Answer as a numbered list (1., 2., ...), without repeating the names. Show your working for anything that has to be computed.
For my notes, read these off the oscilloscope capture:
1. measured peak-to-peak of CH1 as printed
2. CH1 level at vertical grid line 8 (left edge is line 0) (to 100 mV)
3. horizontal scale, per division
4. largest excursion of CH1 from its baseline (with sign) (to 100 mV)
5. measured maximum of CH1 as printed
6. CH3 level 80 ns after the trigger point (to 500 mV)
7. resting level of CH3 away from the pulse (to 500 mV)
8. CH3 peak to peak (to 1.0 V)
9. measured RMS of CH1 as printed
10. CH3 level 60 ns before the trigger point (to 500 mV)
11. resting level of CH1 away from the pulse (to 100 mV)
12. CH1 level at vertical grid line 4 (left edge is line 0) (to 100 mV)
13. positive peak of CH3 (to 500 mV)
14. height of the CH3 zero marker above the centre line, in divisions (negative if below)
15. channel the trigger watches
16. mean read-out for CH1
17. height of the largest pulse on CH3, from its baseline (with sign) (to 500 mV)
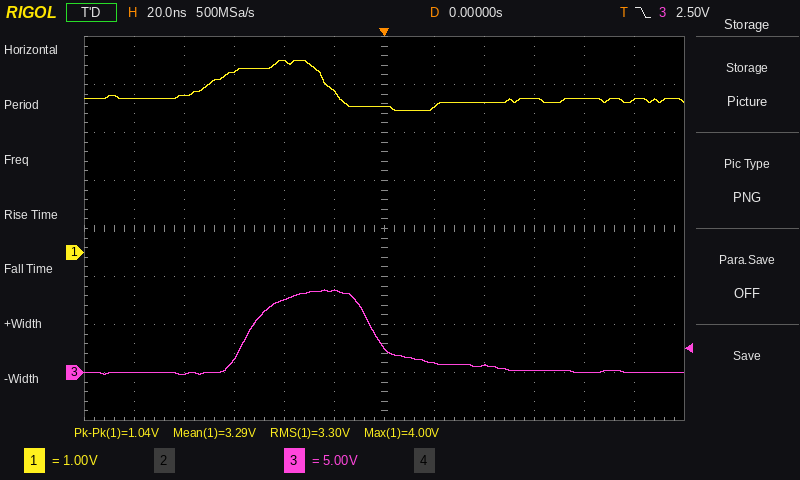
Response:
1. 1.04 V
2. 3.1 V
3. 20 ns
4. +800 mV
5. 4.00 V
6. 0.0 V
7. 0.0 V
8. 9.0 V
9. 3.30 V
10. 1.5 V
11. 3.2 V
12. 4.0 V
13. 8.5 V
14. -3.0 div
15. CH3
16. 3.29 V
17. 8.5 V − (0.0 V) = +8.5 V
